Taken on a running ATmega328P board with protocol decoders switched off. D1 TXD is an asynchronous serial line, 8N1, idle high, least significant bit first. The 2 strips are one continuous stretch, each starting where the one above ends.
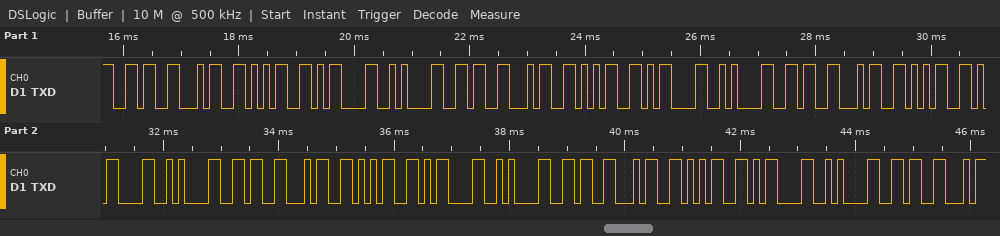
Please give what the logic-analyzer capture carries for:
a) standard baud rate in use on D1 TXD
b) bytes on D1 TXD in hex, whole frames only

9600 baud
36 34 35 0D 0A 36 34 35 0D 0A 36 34 35 0D 0A 36 34 35 0D 0A 36 34 35 0D 0A 36
